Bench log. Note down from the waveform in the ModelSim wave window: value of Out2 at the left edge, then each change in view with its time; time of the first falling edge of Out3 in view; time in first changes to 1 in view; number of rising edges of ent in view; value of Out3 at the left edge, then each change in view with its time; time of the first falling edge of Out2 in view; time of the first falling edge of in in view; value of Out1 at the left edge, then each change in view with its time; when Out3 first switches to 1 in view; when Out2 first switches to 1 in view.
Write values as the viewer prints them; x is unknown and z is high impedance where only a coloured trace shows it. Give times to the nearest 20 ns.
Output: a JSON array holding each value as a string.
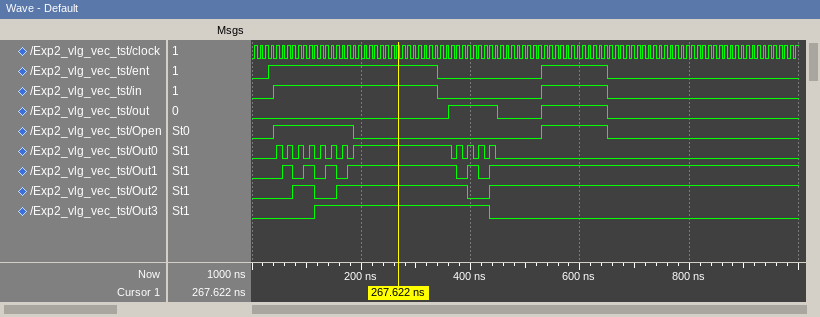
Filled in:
["0, 1 at 80 ns, 0 at 120 ns, 1 at 160 ns, 0 at 400 ns, 1 at 440 ns", "440 ns", "40 ns", "2", "0, 1 at 120 ns, 0 at 440 ns", "120 ns", "340 ns", "0, 1 at 60 ns, 0 at 80 ns, 1 at 100 ns, 0 at 120 ns, 1 at 140 ns, 0 at 160 ns, 1 at 180 ns, 0 at 380 ns, 1 at 400 ns, 0 at 420 ns, 1 at 440 ns", "120 ns", "80 ns"]
